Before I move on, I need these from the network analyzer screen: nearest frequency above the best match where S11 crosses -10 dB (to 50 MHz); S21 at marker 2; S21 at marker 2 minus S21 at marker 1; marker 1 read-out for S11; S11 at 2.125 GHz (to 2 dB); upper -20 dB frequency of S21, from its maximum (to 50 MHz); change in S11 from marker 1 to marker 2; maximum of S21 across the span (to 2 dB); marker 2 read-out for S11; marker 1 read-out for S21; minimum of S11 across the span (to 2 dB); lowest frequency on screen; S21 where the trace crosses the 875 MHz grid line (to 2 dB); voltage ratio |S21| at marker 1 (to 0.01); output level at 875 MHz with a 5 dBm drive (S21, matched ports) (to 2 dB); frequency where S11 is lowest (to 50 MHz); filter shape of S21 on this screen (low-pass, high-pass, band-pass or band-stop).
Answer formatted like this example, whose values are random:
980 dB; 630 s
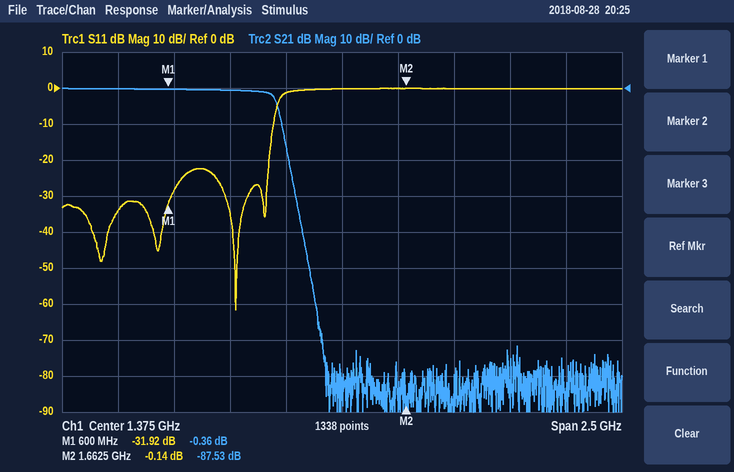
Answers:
1.05 GHz; -87.53 dB; -87.17 dB; -31.92 dB; 0 dB; 1.15 GHz; 31.78 dB; 0 dB; -0.14 dB; -0.36 dB; -62 dB; 125 MHz; 0 dB; 0.96; 4 dBm; 900 MHz; low-pass
